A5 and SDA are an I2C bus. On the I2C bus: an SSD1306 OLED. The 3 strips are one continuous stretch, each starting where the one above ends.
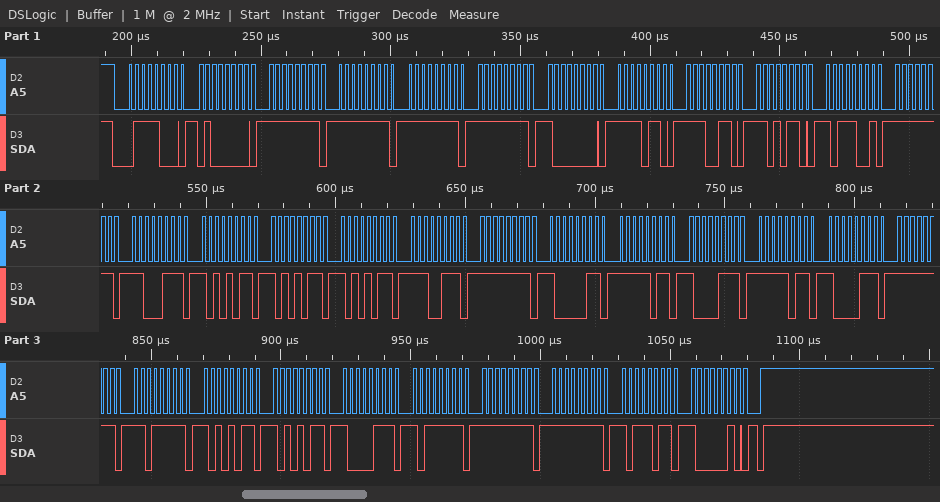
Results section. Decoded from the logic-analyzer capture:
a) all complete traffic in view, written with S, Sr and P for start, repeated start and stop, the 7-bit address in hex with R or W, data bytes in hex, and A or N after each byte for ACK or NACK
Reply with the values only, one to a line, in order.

S 3CW A 40 A FF A FF A FF A FF A 80 A F6 A E6 A D6 A B9 A FF A C7 A AB A AB A AB A E7 A FF A 83 A FB A 87 A FB A 87 A FF A DF A AB A AB A 87 A BF A FF A FF A BB A 82 A P
